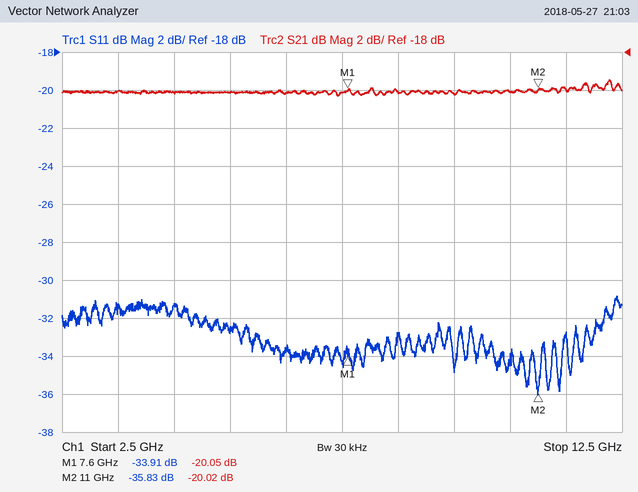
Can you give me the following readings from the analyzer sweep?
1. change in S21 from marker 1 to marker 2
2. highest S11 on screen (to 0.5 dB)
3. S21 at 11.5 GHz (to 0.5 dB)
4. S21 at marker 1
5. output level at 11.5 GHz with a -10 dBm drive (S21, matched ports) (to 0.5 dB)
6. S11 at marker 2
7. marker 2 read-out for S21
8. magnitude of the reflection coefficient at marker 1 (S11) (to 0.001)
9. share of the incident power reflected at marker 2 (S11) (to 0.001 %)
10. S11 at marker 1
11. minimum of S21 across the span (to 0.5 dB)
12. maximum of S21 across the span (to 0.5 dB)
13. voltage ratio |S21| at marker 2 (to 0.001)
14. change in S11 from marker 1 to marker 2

0.03 dB
-31.0 dB
-20.0 dB
-20.05 dB
-30.0 dBm
-35.83 dB
-20.02 dB
0.020
0.026 %
-33.91 dB
-20.5 dB
-19.5 dB
0.100
-1.92 dB
